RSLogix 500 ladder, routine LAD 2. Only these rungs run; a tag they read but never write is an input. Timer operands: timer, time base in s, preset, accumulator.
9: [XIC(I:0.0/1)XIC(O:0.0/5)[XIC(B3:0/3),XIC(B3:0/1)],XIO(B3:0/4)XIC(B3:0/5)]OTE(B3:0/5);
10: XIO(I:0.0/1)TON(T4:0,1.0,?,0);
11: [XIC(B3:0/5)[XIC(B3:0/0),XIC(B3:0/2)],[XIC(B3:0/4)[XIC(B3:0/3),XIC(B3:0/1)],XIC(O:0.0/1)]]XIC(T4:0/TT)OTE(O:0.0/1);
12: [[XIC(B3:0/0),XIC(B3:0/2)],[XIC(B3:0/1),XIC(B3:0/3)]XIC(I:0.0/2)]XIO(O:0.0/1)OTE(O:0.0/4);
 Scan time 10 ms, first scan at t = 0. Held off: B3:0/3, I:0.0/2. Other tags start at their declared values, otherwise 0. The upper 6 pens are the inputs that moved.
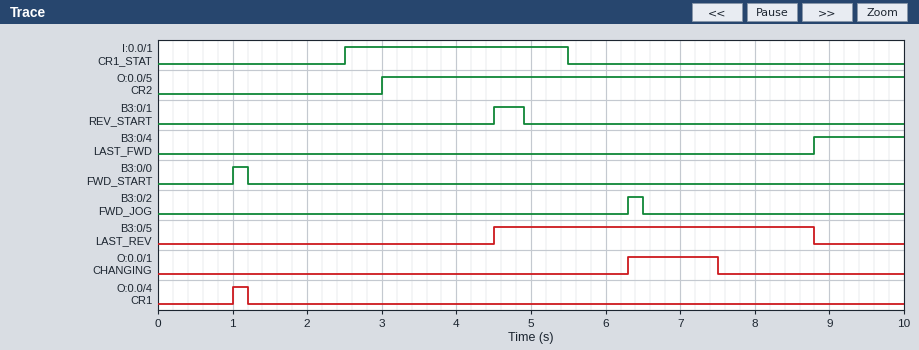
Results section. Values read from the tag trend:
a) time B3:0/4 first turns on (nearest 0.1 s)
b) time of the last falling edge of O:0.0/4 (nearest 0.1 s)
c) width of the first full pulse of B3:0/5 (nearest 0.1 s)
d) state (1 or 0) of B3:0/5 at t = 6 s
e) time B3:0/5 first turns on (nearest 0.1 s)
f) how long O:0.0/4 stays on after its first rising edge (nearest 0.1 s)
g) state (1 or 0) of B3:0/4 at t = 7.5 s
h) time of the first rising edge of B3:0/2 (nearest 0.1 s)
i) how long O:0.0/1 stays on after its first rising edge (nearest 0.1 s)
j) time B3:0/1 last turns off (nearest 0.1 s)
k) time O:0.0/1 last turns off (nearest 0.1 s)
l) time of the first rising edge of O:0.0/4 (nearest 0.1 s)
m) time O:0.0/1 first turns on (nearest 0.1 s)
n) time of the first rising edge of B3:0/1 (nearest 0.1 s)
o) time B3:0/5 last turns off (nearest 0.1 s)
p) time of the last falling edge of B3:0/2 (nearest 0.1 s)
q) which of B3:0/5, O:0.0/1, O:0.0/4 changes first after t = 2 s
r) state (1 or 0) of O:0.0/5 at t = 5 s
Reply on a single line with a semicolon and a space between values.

8.8 s; 1.2 s; 4.3 s; 1; 4.5 s; 0.2 s; 0; 6.3 s; 1.2 s; 4.9 s; 7.5 s; 1.0 s; 6.3 s; 4.5 s; 8.8 s; 6.5 s; B3:0/5; 1
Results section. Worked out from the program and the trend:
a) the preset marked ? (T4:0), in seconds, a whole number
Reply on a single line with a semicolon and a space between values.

2 s
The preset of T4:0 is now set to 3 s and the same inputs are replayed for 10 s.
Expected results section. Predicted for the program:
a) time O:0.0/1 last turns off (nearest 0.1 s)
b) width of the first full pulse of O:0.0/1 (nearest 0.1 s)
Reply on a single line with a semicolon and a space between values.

8.5 s; 2.2 s
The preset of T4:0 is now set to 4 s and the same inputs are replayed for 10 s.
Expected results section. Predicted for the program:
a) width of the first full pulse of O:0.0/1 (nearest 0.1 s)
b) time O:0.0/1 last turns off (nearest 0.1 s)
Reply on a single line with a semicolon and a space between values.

3.2 s; 9.5 s
